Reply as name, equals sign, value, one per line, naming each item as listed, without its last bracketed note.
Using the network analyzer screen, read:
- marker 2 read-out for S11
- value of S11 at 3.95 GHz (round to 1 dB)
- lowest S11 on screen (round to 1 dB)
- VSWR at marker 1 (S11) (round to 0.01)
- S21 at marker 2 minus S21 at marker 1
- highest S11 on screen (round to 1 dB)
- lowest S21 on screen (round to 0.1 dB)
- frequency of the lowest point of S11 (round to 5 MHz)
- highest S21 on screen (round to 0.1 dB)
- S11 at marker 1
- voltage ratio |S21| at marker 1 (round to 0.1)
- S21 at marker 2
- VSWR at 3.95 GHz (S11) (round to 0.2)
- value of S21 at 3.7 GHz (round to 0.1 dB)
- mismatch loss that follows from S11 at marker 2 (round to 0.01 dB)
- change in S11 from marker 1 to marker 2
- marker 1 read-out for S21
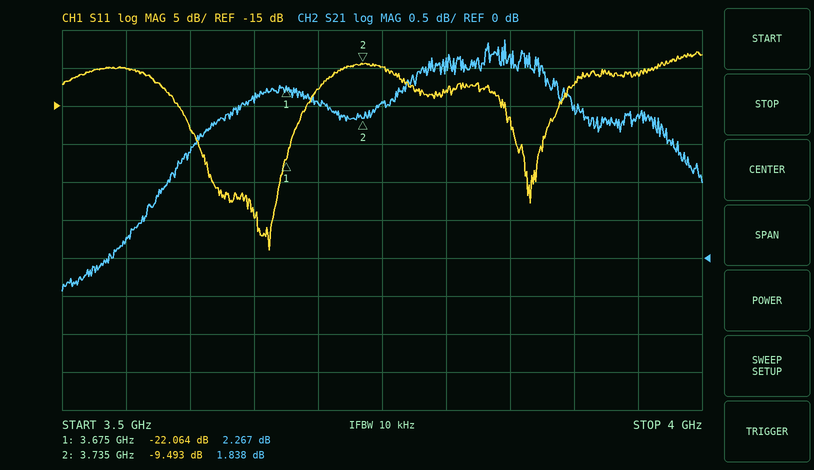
marker 2 read-out for S11 = -9.493 dB
value of S11 at 3.95 GHz = -11 dB
lowest S11 on screen = -34 dB
VSWR at marker 1 (S11) = 1.17
S21 at marker 2 minus S21 at marker 1 = -0.429 dB
highest S11 on screen = -8 dB
lowest S21 on screen = -0.4 dB
frequency of the lowest point of S11 = 3.660 GHz
highest S21 on screen = 2.9 dB
S11 at marker 1 = -22.064 dB
voltage ratio |S21| at marker 1 = 1.3
S21 at marker 2 = 1.838 dB
VSWR at 3.95 GHz (S11) = 1.8
value of S21 at 3.7 GHz = 2.0 dB
mismatch loss that follows from S11 at marker 2 = 0.52 dB
change in S11 from marker 1 to marker 2 = 12.571 dB
marker 1 read-out for S21 = 2.267 dB
